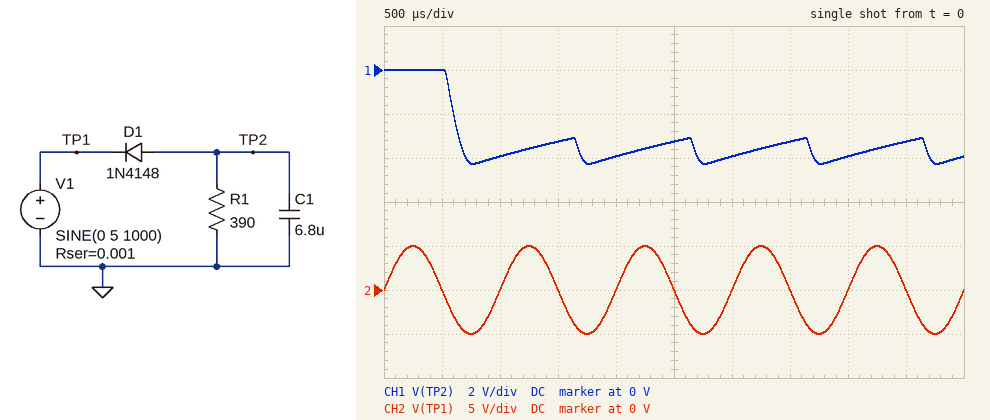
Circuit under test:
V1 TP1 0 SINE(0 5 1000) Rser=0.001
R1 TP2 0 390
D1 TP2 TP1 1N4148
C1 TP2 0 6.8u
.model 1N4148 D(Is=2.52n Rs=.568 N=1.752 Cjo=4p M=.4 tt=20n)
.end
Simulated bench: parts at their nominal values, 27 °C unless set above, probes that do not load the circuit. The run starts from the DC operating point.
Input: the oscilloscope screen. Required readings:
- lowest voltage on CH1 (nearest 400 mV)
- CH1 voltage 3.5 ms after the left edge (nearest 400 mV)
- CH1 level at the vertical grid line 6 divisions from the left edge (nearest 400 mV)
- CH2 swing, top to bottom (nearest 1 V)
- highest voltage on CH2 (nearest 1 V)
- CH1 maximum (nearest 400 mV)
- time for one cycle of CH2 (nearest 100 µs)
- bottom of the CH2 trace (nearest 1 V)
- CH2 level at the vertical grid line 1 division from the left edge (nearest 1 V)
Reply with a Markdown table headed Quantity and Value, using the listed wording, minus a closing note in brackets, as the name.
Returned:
| Quantity | Value |
|---|---|
| lowest voltage on CH1 | -4.4 V |
| CH1 voltage 3.5 ms after the left edge | -3.2 V |
| CH1 level at the vertical grid line 6 divisions from the left edge | -4.0 V |
| CH2 swing, top to bottom | 10 V |
| highest voltage on CH2 | 5 V |
| CH1 maximum | 0 V |
| time for one cycle of CH2 | 1.0 ms |
| bottom of the CH2 trace | -5 V |
| CH2 level at the vertical grid line 1 division from the left edge | 0 V |
